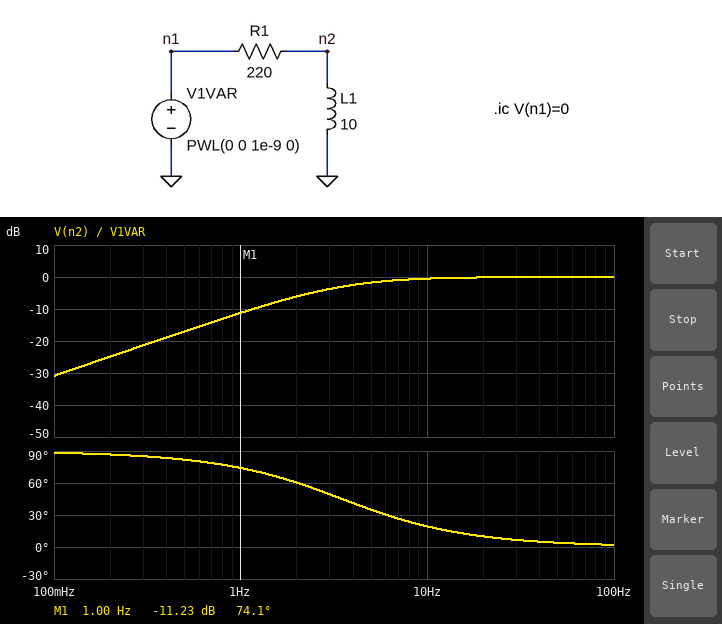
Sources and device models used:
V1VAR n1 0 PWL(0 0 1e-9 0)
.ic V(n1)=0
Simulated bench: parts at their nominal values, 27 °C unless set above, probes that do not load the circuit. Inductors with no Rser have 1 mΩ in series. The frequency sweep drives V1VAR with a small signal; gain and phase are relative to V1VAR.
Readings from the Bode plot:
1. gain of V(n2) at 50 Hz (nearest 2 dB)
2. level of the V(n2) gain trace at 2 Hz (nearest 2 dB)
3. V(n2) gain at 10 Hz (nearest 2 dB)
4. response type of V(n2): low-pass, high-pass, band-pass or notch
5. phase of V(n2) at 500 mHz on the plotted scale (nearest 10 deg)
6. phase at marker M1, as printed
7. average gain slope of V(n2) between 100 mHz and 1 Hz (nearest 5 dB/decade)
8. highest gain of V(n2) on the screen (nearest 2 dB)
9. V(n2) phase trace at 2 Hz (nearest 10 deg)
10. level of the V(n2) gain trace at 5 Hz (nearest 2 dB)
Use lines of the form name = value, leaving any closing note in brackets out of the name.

gain of V(n2) at 50 Hz = 0 dB
level of the V(n2) gain trace at 2 Hz = -6 dB
V(n2) gain at 10 Hz = 0 dB
response type of V(n2): low-pass, high-pass, band-pass or notch = high-pass
phase of V(n2) at 500 mHz on the plotted scale = 80 deg
phase at marker M1, as printed = 74.1 deg
average gain slope of V(n2) between 100 mHz and 1 Hz = 20 dB/decade
highest gain of V(n2) on the screen = 0 dB
V(n2) phase trace at 2 Hz = 60 deg
level of the V(n2) gain trace at 5 Hz = -2 dB
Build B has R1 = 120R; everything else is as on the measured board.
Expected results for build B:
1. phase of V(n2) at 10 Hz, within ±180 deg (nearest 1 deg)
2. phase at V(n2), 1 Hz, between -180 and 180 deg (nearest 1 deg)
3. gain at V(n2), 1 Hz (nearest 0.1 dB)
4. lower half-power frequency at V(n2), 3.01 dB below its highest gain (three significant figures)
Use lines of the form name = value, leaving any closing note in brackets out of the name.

phase of V(n2) at 10 Hz, within ±180 deg = 11 deg
phase at V(n2), 1 Hz, between -180 and 180 deg = 62 deg
gain at V(n2), 1 Hz = -6.7 dB
lower half-power frequency at V(n2), 3.01 dB below its highest gain = 1.91 Hz
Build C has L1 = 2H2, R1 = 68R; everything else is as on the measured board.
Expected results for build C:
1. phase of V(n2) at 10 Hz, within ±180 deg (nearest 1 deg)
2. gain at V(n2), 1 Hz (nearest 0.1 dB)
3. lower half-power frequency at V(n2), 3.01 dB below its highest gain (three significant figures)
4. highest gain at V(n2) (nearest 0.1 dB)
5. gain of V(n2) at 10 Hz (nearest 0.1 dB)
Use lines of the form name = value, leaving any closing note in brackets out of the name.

phase of V(n2) at 10 Hz, within ±180 deg = 26 deg
gain at V(n2), 1 Hz = -14.0 dB
lower half-power frequency at V(n2), 3.01 dB below its highest gain = 4.92 Hz
highest gain at V(n2) = 0 dB
gain of V(n2) at 10 Hz = -0.9 dB
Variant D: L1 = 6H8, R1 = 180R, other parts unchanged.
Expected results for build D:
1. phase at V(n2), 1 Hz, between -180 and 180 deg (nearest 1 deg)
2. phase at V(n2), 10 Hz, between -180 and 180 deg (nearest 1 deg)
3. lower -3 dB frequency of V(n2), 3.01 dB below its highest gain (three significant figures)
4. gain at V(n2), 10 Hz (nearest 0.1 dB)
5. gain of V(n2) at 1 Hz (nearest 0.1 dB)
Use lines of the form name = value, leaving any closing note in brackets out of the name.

phase at V(n2), 1 Hz, between -180 and 180 deg = 77 deg
phase at V(n2), 10 Hz, between -180 and 180 deg = 23 deg
lower -3 dB frequency of V(n2), 3.01 dB below its highest gain = 4.21 Hz
gain at V(n2), 10 Hz = -0.7 dB
gain of V(n2) at 1 Hz = -12.7 dB
